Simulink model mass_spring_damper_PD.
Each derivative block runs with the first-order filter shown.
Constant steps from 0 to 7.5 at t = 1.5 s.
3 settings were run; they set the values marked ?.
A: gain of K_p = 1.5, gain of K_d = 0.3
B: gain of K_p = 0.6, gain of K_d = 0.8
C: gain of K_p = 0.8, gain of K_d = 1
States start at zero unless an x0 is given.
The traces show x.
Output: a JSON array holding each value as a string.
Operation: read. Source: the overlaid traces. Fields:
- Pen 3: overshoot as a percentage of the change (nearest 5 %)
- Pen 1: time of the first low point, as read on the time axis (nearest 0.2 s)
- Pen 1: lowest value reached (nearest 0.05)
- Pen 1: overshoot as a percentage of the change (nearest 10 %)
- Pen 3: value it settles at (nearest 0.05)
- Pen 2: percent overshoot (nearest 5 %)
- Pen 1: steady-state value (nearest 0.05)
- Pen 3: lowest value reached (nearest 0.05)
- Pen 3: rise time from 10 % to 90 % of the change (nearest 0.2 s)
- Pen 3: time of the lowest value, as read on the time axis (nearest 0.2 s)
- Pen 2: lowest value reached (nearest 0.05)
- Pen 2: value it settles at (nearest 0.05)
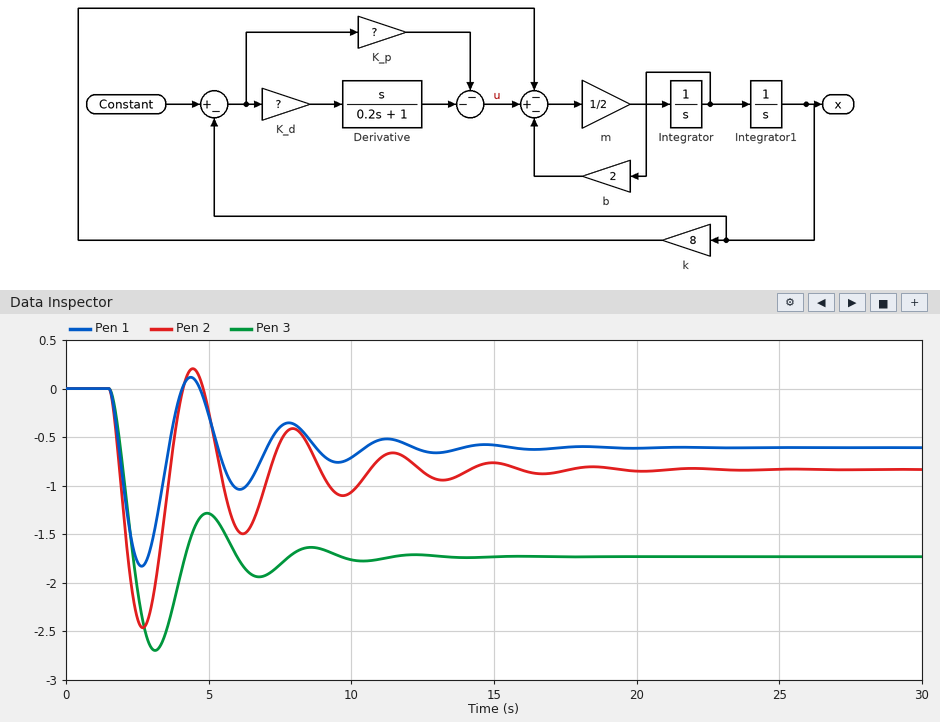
["55 %", "2.6 s", "-1.85", "200 %", "-1.75", "195 %", "-0.60", "-2.70", "0.6 s", "3.2 s", "-2.45", "-0.85"]
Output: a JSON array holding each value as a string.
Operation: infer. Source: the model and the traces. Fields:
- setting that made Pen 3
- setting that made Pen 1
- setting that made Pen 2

["A", "B", "C"]
